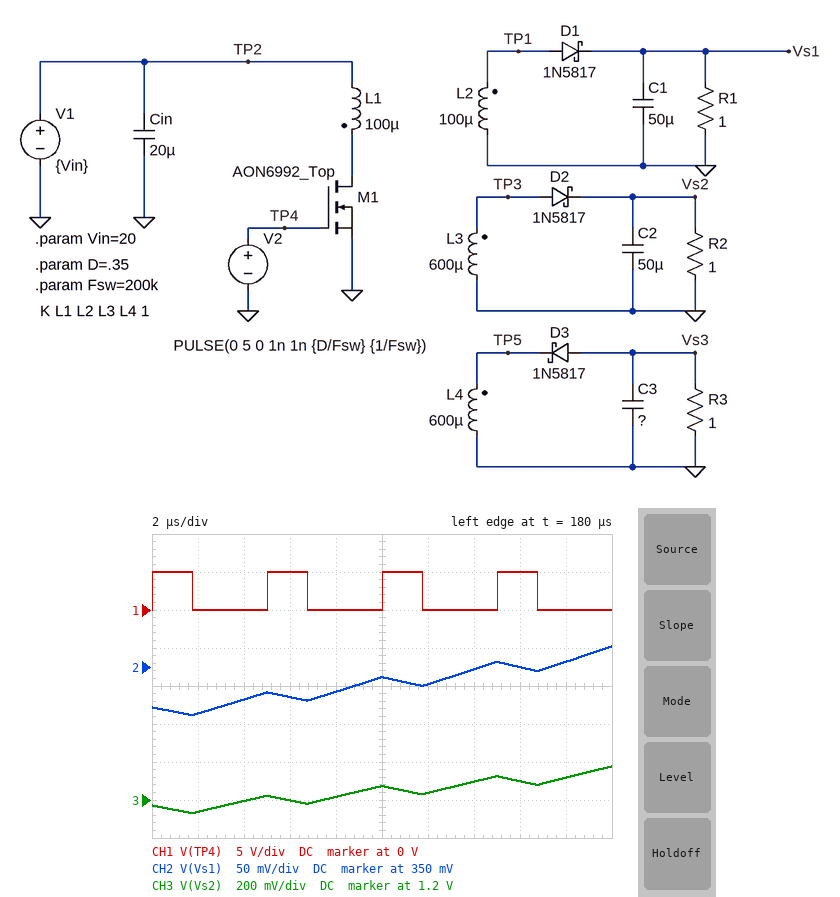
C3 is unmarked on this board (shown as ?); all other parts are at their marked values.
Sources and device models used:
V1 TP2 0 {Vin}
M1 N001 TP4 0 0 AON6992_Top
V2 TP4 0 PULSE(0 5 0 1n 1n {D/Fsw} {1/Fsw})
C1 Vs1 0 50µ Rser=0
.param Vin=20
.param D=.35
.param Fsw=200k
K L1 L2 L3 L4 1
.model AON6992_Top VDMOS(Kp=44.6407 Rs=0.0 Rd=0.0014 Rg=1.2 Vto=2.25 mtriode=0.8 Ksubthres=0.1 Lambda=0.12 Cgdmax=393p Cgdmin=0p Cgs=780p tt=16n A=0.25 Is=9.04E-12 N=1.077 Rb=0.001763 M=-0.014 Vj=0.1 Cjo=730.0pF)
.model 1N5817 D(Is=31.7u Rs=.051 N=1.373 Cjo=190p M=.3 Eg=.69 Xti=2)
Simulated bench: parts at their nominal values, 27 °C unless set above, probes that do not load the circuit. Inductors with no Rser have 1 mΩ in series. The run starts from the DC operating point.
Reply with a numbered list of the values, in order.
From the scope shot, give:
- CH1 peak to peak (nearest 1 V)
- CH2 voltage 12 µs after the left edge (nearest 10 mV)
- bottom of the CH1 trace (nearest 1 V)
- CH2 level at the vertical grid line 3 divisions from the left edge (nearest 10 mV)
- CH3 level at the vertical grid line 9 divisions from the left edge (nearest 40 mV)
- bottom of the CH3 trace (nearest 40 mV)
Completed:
1. 5 V
2. 330 mV
3. 0 V
4. 310 mV
5. 1.32 V
6. 1.12 V
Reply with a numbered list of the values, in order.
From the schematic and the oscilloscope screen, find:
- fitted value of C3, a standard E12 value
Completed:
1. 150 µF
